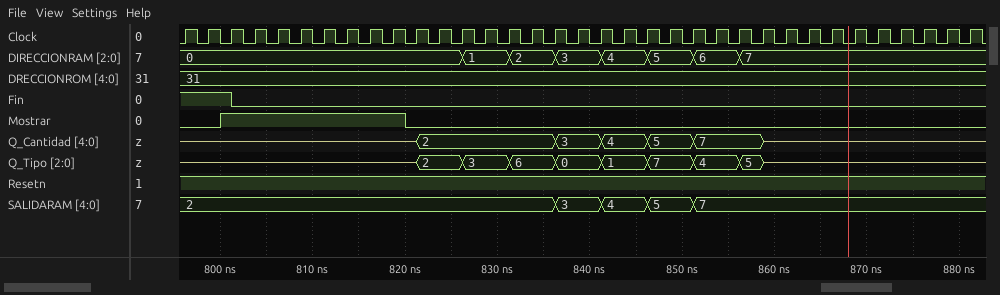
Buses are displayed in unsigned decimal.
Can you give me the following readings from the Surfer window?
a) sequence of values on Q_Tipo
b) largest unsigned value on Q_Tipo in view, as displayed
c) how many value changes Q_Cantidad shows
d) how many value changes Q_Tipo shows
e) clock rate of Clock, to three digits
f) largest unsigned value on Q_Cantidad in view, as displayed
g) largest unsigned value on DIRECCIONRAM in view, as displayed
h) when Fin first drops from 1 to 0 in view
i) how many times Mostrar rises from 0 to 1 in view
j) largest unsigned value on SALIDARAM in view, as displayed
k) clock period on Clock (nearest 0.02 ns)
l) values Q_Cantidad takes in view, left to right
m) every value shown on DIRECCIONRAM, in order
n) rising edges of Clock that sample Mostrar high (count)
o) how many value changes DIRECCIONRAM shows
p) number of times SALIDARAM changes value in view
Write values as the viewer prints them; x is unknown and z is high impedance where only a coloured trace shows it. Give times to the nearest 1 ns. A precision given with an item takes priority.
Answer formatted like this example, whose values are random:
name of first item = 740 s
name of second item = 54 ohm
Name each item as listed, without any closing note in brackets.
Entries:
sequence of values on Q_Tipo = z, 2, 3, 6, 0, 1, 7, 4, 5, z
largest unsigned value on Q_Tipo in view, as displayed = 7
how many value changes Q_Cantidad shows = 6
how many value changes Q_Tipo shows = 9
clock rate of Clock, to three digits = 400 MHz
largest unsigned value on Q_Cantidad in view, as displayed = 7
largest unsigned value on DIRECCIONRAM in view, as displayed = 7
when Fin first drops from 1 to 0 in view = 801 ns
how many times Mostrar rises from 0 to 1 in view = 1
largest unsigned value on SALIDARAM in view, as displayed = 7
clock period on Clock = 2.5 ns
values Q_Cantidad takes in view, left to right = z, 2, 3, 4, 5, 7, z
every value shown on DIRECCIONRAM, in order = 0, 1, 2, 3, 4, 5, 6, 7
rising edges of Clock that sample Mostrar high = 8
how many value changes DIRECCIONRAM shows = 7
number of times SALIDARAM changes value in view = 4
